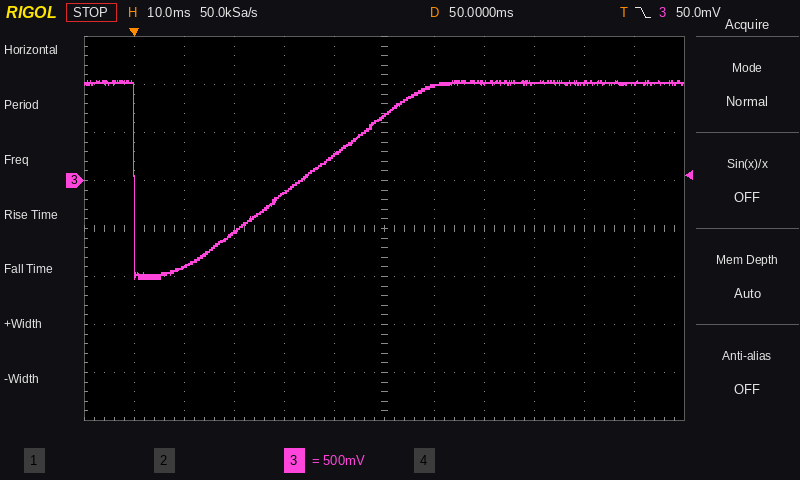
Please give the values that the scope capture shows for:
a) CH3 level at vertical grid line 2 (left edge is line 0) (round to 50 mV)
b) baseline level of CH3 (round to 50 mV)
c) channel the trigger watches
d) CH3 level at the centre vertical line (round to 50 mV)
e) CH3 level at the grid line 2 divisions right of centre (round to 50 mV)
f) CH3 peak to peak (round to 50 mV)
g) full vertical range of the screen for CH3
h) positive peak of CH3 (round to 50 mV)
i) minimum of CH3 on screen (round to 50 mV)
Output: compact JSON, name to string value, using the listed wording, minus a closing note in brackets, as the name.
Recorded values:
{"CH3 level at vertical grid line 2 (left edge is line 0)": "-900 mV", "baseline level of CH3": "1.00 V", "channel the trigger watches": "CH3", "CH3 level at the centre vertical line": "650 mV", "CH3 level at the grid line 2 divisions right of centre": "1.00 V", "CH3 peak to peak": "2.05 V", "full vertical range of the screen for CH3": "4 V", "positive peak of CH3": "1.05 V", "minimum of CH3 on screen": "-1.00 V"}
